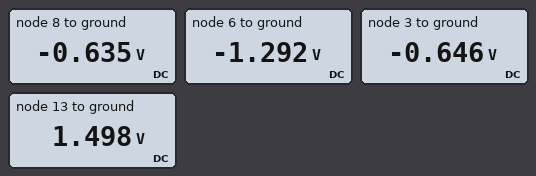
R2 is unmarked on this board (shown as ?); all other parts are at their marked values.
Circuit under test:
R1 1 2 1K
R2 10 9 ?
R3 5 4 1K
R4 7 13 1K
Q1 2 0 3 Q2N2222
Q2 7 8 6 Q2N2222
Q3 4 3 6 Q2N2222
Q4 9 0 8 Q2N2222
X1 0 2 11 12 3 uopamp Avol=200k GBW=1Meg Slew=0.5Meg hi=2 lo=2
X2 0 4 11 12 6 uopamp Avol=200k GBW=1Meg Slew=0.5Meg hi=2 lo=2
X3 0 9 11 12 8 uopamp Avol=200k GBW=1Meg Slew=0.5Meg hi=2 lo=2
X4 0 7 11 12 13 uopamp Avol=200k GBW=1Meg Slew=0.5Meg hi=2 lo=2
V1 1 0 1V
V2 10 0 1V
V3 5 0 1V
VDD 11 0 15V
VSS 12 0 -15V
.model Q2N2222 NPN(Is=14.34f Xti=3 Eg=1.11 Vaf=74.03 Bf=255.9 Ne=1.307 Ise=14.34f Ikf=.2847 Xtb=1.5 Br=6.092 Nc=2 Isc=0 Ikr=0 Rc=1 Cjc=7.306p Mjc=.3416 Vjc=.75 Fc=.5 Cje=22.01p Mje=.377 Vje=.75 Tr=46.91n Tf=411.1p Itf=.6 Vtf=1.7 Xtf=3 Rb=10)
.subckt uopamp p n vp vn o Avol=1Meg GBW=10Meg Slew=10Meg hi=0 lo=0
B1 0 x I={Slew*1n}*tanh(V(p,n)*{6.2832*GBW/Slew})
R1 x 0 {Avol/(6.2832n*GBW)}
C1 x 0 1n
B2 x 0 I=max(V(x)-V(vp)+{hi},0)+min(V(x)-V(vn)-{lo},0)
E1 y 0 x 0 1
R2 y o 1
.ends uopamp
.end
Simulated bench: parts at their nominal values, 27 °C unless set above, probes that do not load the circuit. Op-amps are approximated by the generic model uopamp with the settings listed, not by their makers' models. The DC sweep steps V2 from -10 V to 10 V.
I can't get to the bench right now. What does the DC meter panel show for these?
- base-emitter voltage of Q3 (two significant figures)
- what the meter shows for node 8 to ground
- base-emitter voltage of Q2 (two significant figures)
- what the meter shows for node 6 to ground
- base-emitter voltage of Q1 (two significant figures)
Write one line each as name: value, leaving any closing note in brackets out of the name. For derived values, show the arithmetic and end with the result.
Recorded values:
base-emitter voltage of Q3: -646 mV - (-1.292 V) = 650 mV
what the meter shows for node 8 to ground: -0.635 V
base-emitter voltage of Q2: -635 mV - (-1.292 V) = 660 mV
what the meter shows for node 6 to ground: -1.292 V
base-emitter voltage of Q1: 0 V - (-646 mV) = 650 mV
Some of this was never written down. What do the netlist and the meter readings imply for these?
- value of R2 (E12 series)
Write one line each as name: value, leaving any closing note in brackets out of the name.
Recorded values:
value of R2: 1.5 kΩ
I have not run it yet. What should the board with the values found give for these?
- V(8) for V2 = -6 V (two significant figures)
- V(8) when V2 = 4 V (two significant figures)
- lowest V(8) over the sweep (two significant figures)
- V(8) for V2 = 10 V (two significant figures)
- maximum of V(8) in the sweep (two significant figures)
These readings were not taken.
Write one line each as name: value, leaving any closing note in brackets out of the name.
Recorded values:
V(8) for V2 = -6 V: 12 V
V(8) when V2 = 4 V: -670 mV
lowest V(8) over the sweep: -700 mV
V(8) for V2 = 10 V: -700 mV
maximum of V(8) in the sweep: 12 V
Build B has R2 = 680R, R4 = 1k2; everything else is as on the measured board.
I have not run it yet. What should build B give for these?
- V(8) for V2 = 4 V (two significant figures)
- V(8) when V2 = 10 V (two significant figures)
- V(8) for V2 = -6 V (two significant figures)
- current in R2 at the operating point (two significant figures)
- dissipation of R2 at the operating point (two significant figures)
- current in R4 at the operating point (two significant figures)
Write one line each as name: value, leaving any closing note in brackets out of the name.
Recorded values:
V(8) for V2 = 4 V: -690 mV
V(8) when V2 = 10 V: -720 mV
V(8) for V2 = -6 V: 12 V
current in R2 at the operating point: 1.5 mA
dissipation of R2 at the operating point: 1.5 mW
current in R4 at the operating point: 680 µA
